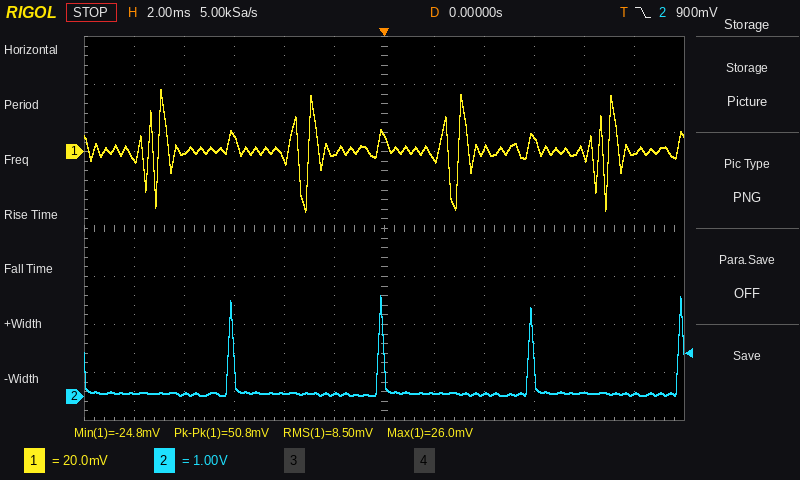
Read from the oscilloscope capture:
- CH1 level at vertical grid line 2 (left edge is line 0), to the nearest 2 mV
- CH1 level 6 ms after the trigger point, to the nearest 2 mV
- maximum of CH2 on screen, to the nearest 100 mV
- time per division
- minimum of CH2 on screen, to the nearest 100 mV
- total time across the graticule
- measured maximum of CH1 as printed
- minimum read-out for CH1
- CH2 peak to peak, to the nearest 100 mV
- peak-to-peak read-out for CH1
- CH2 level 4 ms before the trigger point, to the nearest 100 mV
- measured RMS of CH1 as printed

0 mV
6 mV
2.1 V
2 ms
0.0 V
24 ms
26.0 mV
-24.8 mV
2.1 V
50.8 mV
100 mV
8.50 mV
